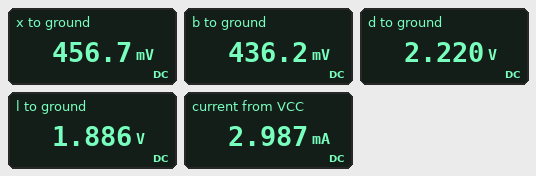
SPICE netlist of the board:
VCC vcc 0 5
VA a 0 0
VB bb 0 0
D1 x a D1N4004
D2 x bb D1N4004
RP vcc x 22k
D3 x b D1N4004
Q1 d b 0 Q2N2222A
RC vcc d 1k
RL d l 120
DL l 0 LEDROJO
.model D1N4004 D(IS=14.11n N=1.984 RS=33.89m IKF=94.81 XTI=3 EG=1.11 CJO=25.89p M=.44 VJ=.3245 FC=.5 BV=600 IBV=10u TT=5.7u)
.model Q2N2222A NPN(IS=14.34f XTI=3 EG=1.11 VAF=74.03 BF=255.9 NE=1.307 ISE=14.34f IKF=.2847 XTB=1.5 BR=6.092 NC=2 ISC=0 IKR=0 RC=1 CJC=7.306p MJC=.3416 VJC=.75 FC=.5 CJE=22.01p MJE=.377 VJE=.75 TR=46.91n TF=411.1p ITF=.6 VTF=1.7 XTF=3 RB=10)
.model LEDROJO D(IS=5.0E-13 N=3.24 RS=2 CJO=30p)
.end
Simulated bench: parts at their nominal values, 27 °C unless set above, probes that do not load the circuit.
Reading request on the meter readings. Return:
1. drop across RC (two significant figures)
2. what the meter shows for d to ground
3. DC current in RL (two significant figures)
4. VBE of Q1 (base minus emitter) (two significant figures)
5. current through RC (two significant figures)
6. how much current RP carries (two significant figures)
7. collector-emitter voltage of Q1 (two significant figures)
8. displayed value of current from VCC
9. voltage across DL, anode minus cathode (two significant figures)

2.8 V
2.220 V
2.8 mA
440 mV
2.8 mA
210 µA
2.2 V
2.987 mA
1.9 V
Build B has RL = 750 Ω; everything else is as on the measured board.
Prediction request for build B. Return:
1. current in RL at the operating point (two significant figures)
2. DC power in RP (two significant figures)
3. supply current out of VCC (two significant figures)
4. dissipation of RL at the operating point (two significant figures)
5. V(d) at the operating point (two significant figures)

1.8 mA
940 µW
2.0 mA
2.4 mW
3.2 V
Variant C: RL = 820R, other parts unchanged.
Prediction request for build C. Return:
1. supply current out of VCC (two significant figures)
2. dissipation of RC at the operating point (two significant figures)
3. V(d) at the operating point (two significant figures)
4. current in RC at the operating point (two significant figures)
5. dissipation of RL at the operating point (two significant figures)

1.9 mA
3.0 mW
3.3 V
1.7 mA
2.5 mW
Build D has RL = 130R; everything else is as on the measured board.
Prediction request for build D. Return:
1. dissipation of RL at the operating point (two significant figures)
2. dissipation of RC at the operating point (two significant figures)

990 µW
7.6 mW
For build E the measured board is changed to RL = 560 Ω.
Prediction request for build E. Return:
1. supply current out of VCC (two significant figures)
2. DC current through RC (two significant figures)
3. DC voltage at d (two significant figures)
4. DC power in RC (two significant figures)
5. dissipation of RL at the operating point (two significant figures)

2.2 mA
2.0 mA
3.0 V
4.1 mW
2.3 mW
